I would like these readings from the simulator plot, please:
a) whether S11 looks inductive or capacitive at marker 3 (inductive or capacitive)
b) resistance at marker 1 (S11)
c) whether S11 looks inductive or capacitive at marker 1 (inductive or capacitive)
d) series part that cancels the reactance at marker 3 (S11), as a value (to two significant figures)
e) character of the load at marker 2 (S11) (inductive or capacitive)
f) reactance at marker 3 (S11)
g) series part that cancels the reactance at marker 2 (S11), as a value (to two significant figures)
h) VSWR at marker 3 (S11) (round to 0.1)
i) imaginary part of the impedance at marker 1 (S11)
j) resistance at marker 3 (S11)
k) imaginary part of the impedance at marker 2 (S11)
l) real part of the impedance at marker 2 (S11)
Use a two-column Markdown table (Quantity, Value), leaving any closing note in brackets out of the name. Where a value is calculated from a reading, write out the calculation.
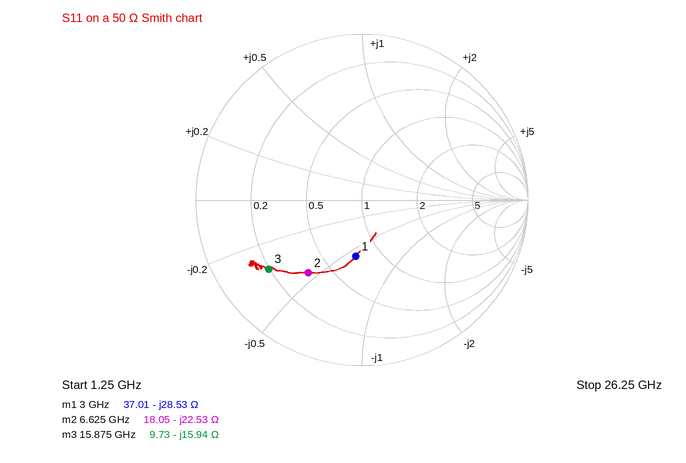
| Quantity | Value |
|---|---|
| whether S11 looks inductive or capacitive at marker 3 | capacitive |
| resistance at marker 1 | 37.01 Ω |
| whether S11 looks inductive or capacitive at marker 1 | capacitive |
| series part that cancels the reactance at marker 3 (S11), as a value | L = 15.94 Ω/(2π × 15.875 GHz) ≈ 160 pH |
| character of the load at marker 2 (S11) | capacitive |
| reactance at marker 3 | -15.94 Ω |
| series part that cancels the reactance at marker 2 (S11), as a value | L = 22.53 Ω/(2π × 6.625 GHz) ≈ 541 pH, so 540 pH to two significant figures |
| VSWR at marker 3 (S11) | 5.7 |
| imaginary part of the impedance at marker 1 | -28.53 Ω |
| resistance at marker 3 | 9.73 Ω |
| imaginary part of the impedance at marker 2 | -22.53 Ω |
| real part of the impedance at marker 2 | 18.05 Ω |
